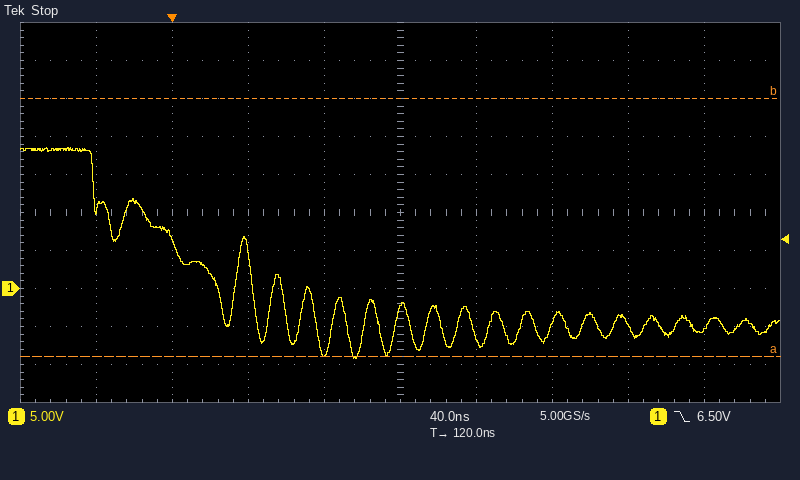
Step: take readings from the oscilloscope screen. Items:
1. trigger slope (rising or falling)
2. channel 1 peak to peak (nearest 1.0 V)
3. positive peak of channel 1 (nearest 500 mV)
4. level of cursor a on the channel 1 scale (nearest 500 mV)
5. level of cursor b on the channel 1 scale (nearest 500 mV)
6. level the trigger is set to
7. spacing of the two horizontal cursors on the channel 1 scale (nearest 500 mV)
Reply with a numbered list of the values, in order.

1. falling
2. 28.0 V
3. 18.5 V
4. -9.0 V
5. 25.0 V
6. 6.50 V
7. 34.0 V
